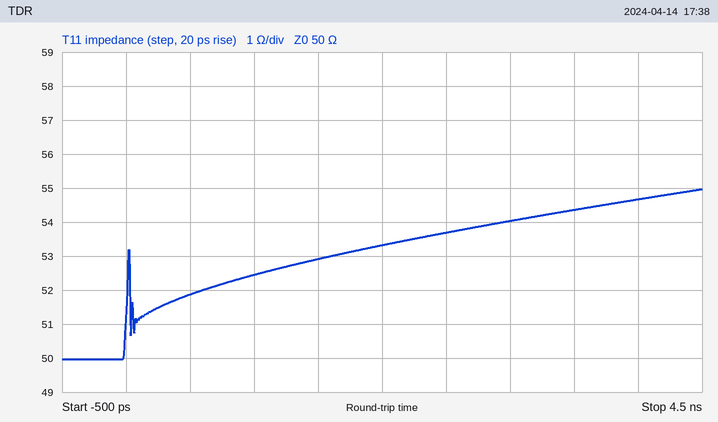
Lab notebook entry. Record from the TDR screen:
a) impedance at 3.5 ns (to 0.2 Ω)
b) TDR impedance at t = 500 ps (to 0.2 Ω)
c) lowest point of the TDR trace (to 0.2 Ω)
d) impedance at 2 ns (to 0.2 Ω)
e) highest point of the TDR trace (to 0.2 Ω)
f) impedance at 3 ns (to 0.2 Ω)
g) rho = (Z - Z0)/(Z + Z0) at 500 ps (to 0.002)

54.4 Ω
51.8 Ω
50.0 Ω
53.4 Ω
55.0 Ω
54.0 Ω
+0.018
